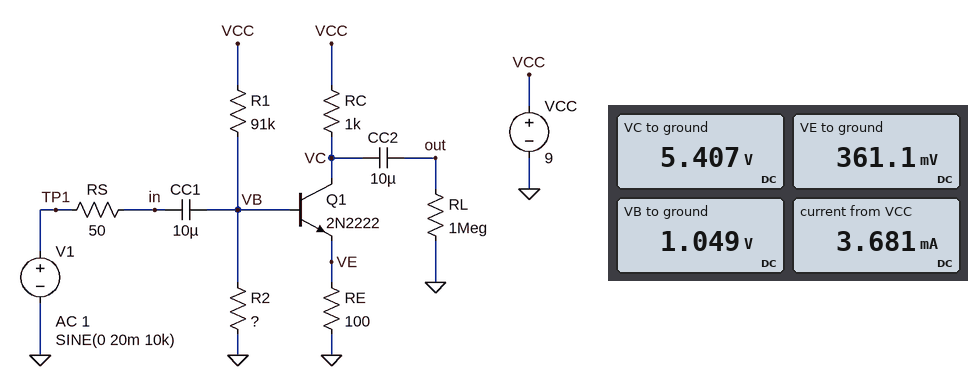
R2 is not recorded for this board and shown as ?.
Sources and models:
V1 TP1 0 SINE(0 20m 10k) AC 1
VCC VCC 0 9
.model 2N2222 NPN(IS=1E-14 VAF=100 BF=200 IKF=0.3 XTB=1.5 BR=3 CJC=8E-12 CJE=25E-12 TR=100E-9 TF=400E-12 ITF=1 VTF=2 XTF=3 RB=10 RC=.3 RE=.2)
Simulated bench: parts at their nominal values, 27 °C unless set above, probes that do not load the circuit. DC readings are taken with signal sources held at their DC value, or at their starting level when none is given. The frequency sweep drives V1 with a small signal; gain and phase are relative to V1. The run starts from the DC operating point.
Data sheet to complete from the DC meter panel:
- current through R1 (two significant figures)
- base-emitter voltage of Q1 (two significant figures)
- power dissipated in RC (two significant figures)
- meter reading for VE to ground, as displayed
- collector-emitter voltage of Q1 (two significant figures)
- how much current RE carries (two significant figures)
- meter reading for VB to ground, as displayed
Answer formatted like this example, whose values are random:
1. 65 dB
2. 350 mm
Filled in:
1. 87 µA
2. 690 mV
3. 13 mW
4. 361.1 mV
5. 5.0 V
6. 3.6 mA
7. 1.049 V
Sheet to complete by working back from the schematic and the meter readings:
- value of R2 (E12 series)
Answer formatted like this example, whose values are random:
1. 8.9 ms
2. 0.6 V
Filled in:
1. 15 kΩ
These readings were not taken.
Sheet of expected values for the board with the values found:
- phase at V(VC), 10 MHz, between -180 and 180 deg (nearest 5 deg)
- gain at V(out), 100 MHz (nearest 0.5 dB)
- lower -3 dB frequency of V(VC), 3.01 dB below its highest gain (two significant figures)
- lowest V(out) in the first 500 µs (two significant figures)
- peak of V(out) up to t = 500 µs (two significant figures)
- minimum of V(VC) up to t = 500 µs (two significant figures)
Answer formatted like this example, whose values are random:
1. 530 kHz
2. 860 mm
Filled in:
1. 150 deg
2. 6.5 dB
3. 2.0 Hz
4. -180 mV
5. 180 mV
6. 5.2 V
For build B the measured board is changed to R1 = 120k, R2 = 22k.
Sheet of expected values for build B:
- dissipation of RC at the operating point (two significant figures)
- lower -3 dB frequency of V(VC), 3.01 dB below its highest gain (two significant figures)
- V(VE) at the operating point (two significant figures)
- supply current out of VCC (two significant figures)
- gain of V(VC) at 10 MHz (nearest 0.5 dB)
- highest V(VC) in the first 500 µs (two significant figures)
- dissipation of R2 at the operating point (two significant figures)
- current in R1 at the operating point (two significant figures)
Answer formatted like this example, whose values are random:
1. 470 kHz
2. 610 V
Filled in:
1. 14 mW
2. 1.6 Hz
3. 370 mV
4. 3.8 mA
5. 18.5 dB
6. 5.5 V
7. 51 µW
8. 66 µA
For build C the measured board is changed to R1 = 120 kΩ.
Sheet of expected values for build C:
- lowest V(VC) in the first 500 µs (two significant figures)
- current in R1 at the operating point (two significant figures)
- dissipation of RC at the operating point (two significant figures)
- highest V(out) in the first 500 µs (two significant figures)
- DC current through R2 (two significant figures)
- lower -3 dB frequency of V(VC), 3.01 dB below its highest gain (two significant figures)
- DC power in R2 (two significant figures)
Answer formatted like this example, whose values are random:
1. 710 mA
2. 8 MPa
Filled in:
1. 6.8 V
2. 68 µA
3. 4.0 mW
4. 170 mV
5. 58 µA
6. 1.9 Hz
7. 51 µW
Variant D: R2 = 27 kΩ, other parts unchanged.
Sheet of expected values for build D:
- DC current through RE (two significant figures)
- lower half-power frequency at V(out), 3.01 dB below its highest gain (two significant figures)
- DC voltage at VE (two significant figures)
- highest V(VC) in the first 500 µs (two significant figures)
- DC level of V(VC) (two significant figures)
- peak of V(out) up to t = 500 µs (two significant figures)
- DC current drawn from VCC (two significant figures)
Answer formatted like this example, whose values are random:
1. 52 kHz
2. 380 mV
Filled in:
1. 6.6 mA
2. 1.6 Hz
3. 660 mV
4. 2.6 V
5. 2.4 V
6. 190 mV
7. 6.7 mA
